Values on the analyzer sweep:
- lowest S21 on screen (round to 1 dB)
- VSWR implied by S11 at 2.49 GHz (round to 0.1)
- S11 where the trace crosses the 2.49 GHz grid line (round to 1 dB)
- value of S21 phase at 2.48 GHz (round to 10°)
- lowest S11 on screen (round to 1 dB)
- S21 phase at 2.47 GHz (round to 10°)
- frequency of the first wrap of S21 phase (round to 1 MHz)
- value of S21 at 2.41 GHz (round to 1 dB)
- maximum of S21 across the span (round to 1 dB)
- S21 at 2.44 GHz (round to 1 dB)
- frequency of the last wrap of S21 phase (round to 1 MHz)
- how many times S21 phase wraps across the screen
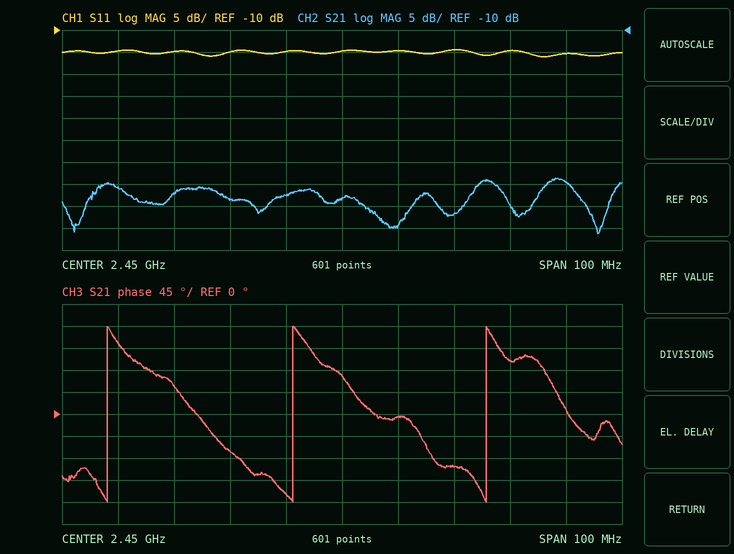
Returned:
-56 dB
1.4
-15 dB
110°
-16 dB
-110°
2.408 GHz
-46 dB
-44 dB
-48 dB
2.476 GHz
3
